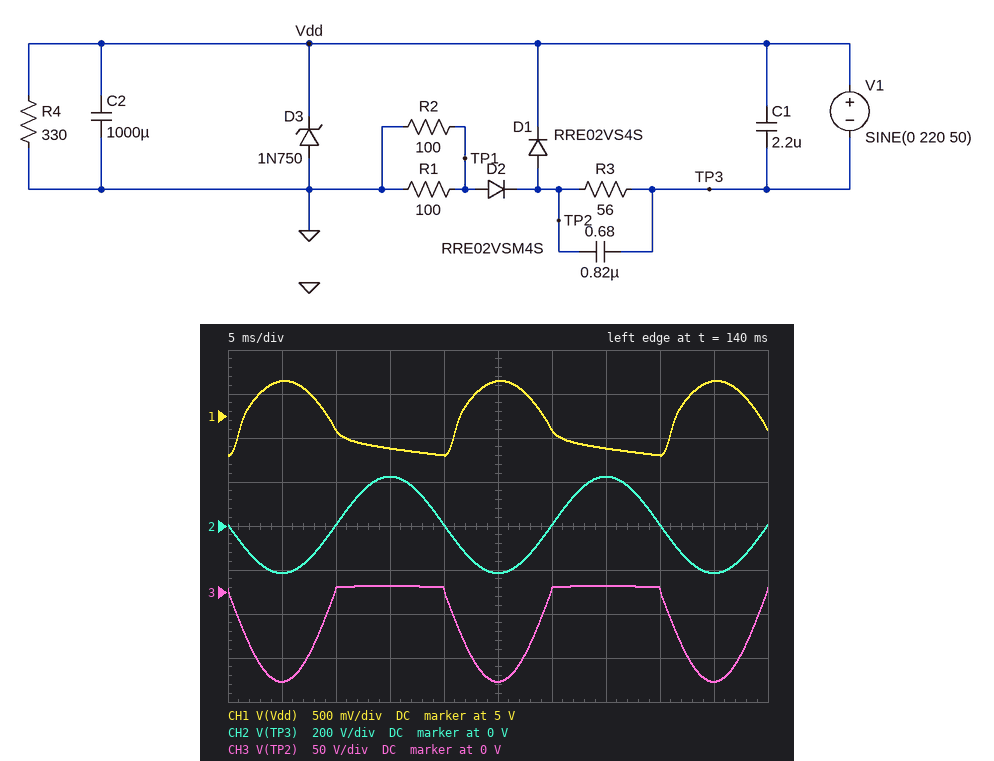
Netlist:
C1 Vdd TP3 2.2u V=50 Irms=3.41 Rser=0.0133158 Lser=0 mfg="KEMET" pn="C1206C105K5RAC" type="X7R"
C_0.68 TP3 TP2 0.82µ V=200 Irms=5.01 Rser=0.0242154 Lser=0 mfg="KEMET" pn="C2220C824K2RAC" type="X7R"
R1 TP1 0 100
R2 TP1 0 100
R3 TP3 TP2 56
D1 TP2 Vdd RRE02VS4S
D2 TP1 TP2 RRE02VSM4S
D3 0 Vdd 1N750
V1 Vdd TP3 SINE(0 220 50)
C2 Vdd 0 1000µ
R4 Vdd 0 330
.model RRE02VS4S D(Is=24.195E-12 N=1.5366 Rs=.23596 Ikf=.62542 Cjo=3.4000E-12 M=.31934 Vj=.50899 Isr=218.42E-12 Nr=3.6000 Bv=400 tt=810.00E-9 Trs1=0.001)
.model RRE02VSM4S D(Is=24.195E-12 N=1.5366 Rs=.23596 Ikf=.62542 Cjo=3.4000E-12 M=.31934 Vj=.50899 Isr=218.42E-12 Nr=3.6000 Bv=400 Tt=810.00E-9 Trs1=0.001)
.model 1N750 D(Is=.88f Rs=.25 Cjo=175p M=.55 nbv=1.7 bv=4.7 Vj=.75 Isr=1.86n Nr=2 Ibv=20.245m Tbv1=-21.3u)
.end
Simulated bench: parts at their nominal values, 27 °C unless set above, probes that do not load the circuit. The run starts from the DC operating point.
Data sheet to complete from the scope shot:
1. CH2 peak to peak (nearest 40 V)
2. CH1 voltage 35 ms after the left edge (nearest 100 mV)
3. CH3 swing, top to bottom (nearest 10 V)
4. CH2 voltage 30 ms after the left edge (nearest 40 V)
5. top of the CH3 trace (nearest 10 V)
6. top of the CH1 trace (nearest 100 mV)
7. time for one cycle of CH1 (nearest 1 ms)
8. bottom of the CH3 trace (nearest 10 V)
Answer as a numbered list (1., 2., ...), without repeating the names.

1. 440 V
2. 4.6 V
3. 110 V
4. 0 V
5. 10 V
6. 5.4 V
7. 20 ms
8. -100 V
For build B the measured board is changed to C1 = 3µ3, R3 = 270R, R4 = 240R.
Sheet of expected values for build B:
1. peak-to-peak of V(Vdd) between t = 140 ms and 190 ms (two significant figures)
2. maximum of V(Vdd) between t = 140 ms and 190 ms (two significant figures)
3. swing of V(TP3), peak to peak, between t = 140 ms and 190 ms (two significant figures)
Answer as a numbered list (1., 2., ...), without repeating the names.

1. 510 mV
2. 5.0 V
3. 440 V
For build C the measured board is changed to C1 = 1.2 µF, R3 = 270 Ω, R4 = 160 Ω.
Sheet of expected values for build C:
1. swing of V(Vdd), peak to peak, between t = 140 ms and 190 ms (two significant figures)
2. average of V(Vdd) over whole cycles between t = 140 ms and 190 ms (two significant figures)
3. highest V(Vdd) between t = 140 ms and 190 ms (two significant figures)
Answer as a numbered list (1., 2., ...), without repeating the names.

1. 590 mV
2. 4.7 V
3. 5.0 V
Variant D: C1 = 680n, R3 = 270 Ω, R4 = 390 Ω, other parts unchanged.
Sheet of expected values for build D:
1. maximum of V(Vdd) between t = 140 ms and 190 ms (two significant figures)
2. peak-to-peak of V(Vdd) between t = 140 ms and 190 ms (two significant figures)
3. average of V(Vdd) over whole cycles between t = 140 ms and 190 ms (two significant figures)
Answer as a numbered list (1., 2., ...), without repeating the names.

1. 5.0 V
2. 460 mV
3. 4.8 V
